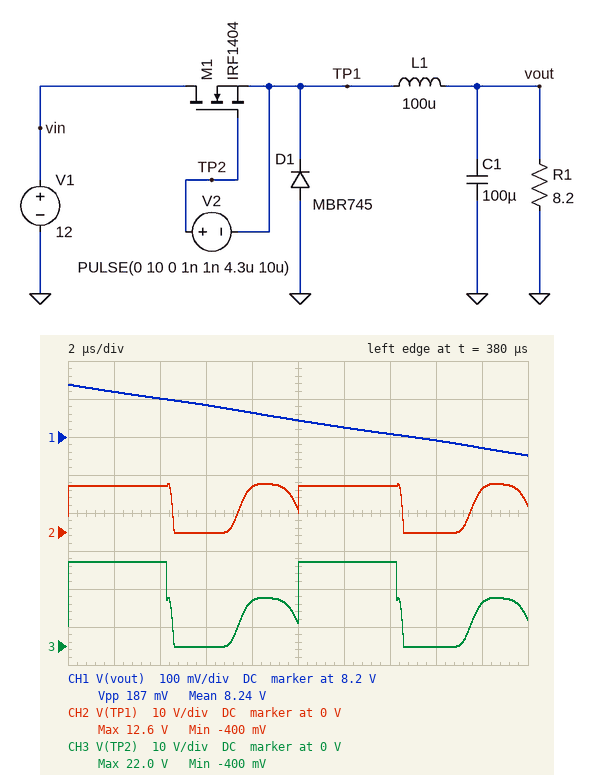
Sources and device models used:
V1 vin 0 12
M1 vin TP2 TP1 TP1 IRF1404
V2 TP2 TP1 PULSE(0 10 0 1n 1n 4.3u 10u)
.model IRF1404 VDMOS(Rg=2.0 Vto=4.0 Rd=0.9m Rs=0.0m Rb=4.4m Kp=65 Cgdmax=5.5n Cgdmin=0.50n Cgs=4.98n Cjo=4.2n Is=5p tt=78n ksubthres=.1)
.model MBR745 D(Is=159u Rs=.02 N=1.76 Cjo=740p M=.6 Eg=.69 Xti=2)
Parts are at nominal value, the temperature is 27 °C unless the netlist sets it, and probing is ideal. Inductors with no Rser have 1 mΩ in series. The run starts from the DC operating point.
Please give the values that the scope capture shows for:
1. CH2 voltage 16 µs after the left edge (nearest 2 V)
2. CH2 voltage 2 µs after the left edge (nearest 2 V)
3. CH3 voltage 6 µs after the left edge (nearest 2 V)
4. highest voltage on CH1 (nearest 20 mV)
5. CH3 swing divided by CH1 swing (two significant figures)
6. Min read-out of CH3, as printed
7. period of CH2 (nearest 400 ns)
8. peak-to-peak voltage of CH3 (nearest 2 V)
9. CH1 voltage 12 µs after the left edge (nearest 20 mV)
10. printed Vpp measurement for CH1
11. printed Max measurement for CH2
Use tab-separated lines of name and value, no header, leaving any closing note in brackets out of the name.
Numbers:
CH2 voltage 16 µs after the left edge	0 V
CH2 voltage 2 µs after the left edge	12 V
CH3 voltage 6 µs after the left edge	0 V
highest voltage on CH1	8.34 V
CH3 swing divided by CH1 swing	120
Min read-out of CH3, as printed	-400 mV
period of CH2	10.0 µs
peak-to-peak voltage of CH3	22 V
CH1 voltage 12 µs after the left edge	8.22 V
printed Vpp measurement for CH1	187 mV
printed Max measurement for CH2	12.6 V
